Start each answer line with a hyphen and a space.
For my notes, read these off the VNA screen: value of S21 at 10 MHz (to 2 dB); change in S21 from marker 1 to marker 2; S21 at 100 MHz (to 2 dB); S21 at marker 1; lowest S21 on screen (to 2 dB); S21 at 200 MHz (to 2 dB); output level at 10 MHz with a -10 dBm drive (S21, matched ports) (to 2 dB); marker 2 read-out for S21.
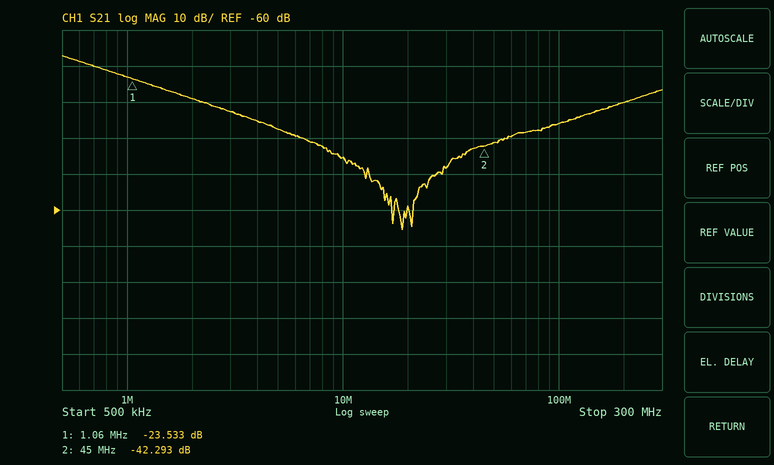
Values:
- -46 dB
- -18.760 dB
- -36 dB
- -23.533 dB
- -66 dB
- -30 dB
- -56 dBm
- -42.293 dB
